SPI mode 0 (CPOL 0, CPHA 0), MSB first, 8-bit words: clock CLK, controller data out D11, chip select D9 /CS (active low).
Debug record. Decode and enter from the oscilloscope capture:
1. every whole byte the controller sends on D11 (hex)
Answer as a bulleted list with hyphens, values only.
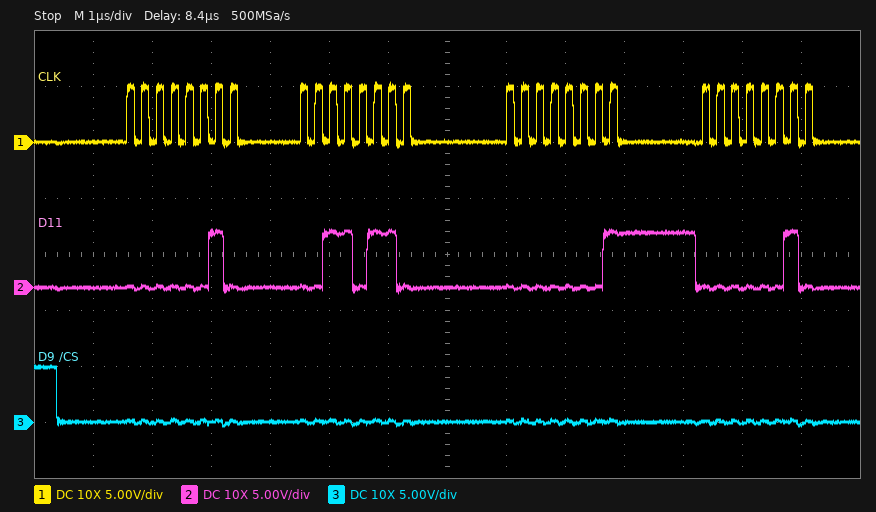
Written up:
- 02 36 01 02
